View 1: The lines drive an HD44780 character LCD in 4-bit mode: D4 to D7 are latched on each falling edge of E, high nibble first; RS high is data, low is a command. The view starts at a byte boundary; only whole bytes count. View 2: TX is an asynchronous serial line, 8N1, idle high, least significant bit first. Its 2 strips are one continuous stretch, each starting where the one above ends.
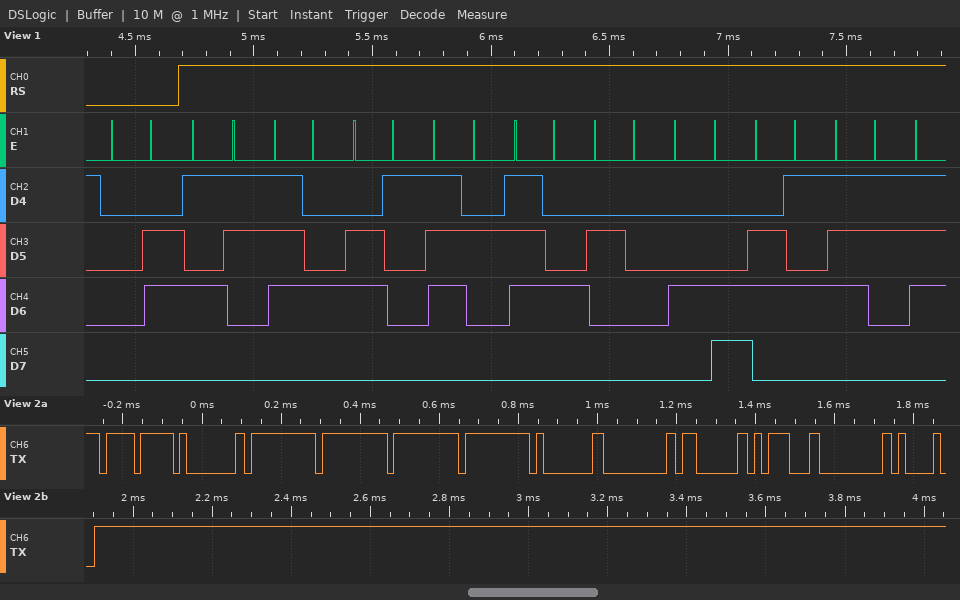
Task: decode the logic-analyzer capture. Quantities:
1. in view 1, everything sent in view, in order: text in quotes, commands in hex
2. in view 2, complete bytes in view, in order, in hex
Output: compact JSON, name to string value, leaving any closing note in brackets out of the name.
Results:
{"in view 1, everything sent in view, in order: text in quotes, commands in hex": "0x06 \"Start Les\"", "in view 2, complete bytes in view, in order, in hex": "EF 01 FF FF FF FF 01 00 03 1D 00 21"}
